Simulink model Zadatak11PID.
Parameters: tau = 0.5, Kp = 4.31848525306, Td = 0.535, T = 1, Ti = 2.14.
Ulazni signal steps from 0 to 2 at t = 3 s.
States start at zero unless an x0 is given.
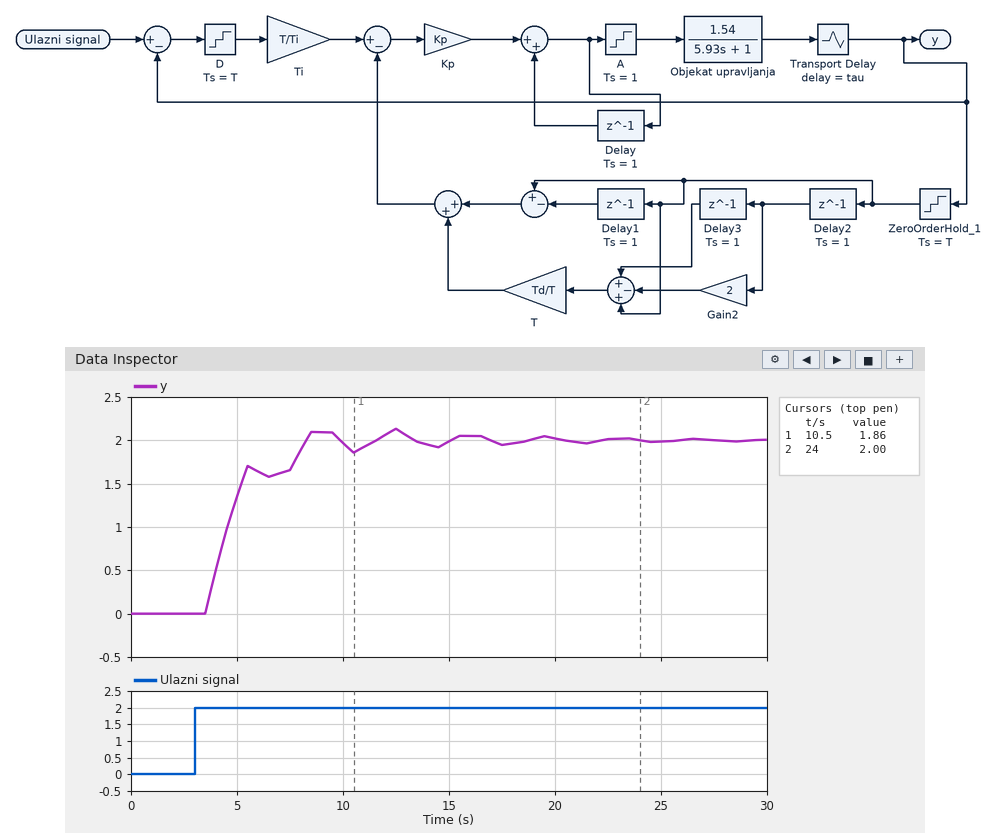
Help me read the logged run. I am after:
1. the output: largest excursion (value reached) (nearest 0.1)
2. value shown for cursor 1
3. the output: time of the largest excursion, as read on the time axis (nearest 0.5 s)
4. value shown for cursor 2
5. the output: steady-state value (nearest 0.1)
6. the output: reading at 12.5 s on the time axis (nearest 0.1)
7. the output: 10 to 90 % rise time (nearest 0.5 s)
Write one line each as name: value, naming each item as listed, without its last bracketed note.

the output: largest excursion (value reached): 2.1
value shown for cursor 1: 1.86
the output: time of the largest excursion, as read on the time axis: 12.5 s
value shown for cursor 2: 2.00
the output: steady-state value: 2.0
the output: reading at 12.5 s on the time axis: 2.1
the output: 10 to 90 % rise time: 4.0 s
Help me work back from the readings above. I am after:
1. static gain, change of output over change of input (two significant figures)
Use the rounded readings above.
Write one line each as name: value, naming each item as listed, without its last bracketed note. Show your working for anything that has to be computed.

static gain, change of output over change of input: (2 - 0) / (2 - 0) = 1.0
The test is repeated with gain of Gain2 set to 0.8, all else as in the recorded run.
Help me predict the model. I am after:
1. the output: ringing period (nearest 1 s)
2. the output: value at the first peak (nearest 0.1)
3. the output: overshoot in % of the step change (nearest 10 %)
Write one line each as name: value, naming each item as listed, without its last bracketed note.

the output: ringing period: 5 s
the output: value at the first peak: 1.7
the output: overshoot in % of the step change: 100 %
